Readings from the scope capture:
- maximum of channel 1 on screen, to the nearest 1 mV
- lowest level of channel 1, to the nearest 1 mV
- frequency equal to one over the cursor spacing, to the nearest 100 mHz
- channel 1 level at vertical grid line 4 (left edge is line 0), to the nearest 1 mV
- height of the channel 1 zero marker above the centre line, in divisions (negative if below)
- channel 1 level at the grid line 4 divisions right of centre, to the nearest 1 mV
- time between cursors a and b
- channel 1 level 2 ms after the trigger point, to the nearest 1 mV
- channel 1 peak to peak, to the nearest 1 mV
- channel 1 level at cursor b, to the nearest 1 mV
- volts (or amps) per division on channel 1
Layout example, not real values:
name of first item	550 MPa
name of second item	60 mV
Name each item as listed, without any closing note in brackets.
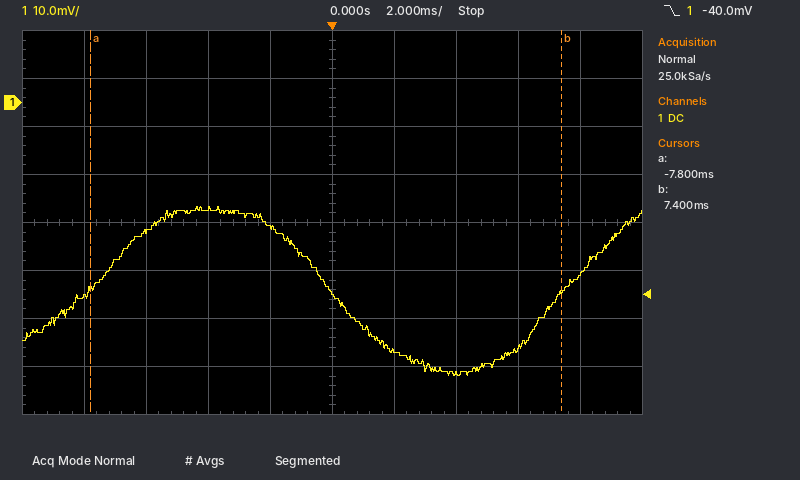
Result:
maximum of channel 1 on screen, to the nearest 1 mV	-22 mV
lowest level of channel 1, to the nearest 1 mV	-57 mV
frequency equal to one over the cursor spacing, to the nearest 100 mHz	65.8 Hz
channel 1 level at vertical grid line 4 (left edge is line 0), to the nearest 1 mV	-26 mV
height of the channel 1 zero marker above the centre line, in divisions	+2.5 div
channel 1 level at the grid line 4 divisions right of centre, to the nearest 1 mV	-36 mV
time between cursors a and b	15.2 ms
channel 1 level 2 ms after the trigger point, to the nearest 1 mV	-52 mV
channel 1 peak to peak, to the nearest 1 mV	35 mV
channel 1 level at cursor b, to the nearest 1 mV	-39 mV
volts (or amps) per division on channel 1	10 mV
